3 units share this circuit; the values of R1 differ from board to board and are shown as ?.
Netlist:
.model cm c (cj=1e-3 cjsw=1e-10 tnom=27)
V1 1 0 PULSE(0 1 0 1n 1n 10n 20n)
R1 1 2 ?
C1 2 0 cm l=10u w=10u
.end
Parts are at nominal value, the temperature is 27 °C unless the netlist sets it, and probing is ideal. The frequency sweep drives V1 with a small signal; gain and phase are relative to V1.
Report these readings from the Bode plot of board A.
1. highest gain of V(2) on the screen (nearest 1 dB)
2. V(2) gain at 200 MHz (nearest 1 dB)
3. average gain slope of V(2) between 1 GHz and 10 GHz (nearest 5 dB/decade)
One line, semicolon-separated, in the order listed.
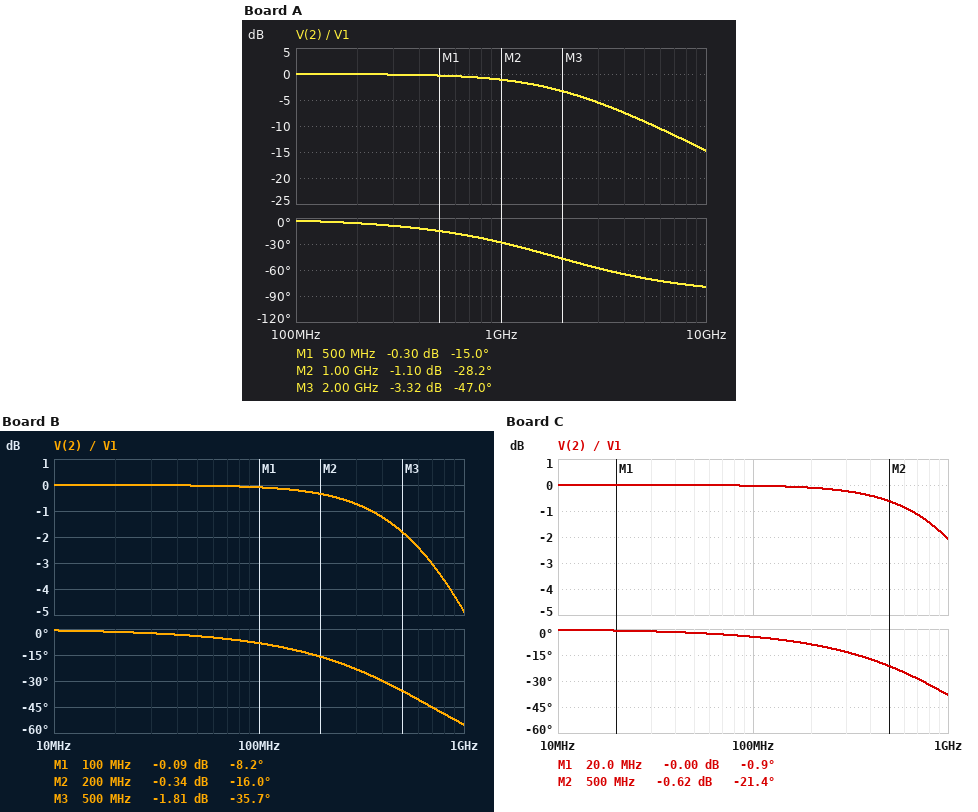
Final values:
0 dB; 0 dB; -15 dB/decade
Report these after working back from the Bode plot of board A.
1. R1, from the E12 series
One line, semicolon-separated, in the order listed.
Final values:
820 Ω
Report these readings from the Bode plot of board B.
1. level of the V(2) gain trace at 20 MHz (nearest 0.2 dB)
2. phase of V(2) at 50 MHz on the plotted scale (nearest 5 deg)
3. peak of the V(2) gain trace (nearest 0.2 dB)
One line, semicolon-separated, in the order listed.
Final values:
0 dB; -5 deg; 0 dB
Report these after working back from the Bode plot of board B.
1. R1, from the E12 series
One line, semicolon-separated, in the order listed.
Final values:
2.2 kΩ
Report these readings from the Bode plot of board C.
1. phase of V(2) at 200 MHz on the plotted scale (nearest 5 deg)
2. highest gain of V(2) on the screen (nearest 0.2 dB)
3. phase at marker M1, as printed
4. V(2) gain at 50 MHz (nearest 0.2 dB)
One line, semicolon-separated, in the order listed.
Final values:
-10 deg; 0 dB; -0.9 deg; 0 dB
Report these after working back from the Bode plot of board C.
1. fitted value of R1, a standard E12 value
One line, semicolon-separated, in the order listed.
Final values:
1.2 kΩ
